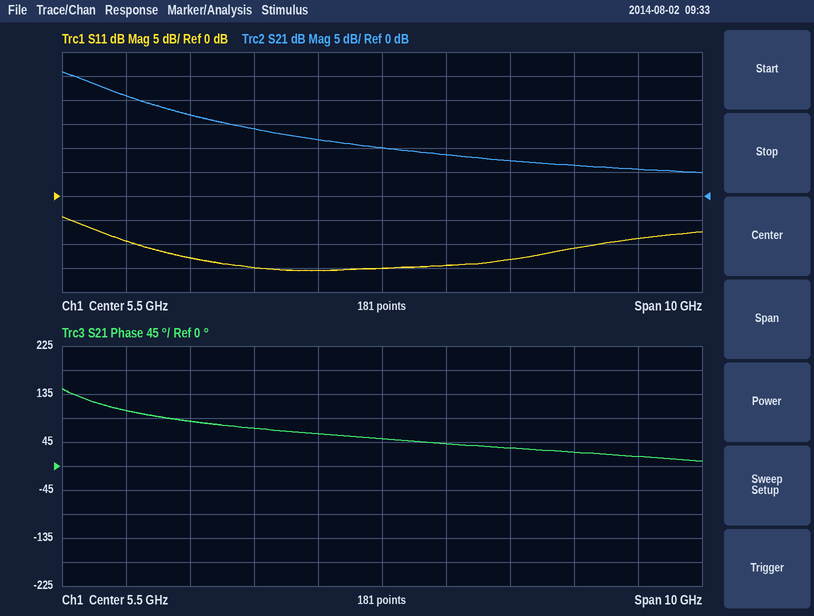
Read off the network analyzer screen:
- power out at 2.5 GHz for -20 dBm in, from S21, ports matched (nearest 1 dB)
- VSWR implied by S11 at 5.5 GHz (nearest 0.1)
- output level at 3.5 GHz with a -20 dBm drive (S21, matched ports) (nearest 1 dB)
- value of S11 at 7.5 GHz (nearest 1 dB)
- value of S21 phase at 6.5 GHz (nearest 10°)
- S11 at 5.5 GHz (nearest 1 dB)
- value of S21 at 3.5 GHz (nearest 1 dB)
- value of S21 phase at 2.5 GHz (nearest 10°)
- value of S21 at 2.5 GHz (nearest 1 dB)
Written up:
-3 dBm
1.4
-6 dBm
-13 dB
40°
-15 dB
14 dB
80°
17 dB
